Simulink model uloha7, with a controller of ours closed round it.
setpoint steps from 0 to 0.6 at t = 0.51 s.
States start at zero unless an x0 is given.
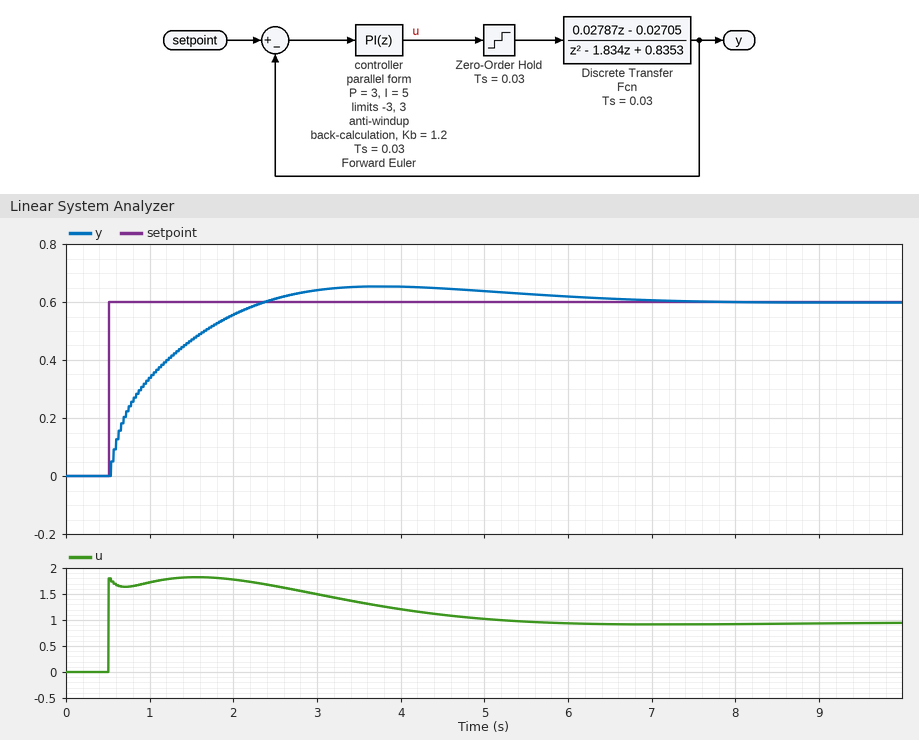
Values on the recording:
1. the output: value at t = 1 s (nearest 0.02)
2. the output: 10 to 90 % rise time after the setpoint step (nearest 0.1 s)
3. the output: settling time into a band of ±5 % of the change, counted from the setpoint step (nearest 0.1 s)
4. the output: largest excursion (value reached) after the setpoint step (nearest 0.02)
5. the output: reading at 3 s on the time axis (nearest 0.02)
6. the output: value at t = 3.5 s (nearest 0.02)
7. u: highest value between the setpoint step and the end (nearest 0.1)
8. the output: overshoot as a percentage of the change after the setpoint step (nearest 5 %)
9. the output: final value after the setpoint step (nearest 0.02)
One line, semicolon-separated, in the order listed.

0.34; 1.3 s; 4.9 s; 0.66; 0.64; 0.66; 1.8; 10 %; 0.60
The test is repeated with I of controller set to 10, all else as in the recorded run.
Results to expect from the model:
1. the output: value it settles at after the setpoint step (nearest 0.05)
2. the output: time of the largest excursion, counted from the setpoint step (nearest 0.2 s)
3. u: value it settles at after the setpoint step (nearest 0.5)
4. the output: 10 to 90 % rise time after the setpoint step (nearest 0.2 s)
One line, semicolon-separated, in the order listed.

0.60; 2.0 s; 1.0; 0.8 s
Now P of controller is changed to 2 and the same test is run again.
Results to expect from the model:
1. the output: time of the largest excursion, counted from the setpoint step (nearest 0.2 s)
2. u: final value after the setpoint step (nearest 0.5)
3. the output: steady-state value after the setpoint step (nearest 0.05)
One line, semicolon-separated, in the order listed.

3.0 s; 1.0; 0.60
